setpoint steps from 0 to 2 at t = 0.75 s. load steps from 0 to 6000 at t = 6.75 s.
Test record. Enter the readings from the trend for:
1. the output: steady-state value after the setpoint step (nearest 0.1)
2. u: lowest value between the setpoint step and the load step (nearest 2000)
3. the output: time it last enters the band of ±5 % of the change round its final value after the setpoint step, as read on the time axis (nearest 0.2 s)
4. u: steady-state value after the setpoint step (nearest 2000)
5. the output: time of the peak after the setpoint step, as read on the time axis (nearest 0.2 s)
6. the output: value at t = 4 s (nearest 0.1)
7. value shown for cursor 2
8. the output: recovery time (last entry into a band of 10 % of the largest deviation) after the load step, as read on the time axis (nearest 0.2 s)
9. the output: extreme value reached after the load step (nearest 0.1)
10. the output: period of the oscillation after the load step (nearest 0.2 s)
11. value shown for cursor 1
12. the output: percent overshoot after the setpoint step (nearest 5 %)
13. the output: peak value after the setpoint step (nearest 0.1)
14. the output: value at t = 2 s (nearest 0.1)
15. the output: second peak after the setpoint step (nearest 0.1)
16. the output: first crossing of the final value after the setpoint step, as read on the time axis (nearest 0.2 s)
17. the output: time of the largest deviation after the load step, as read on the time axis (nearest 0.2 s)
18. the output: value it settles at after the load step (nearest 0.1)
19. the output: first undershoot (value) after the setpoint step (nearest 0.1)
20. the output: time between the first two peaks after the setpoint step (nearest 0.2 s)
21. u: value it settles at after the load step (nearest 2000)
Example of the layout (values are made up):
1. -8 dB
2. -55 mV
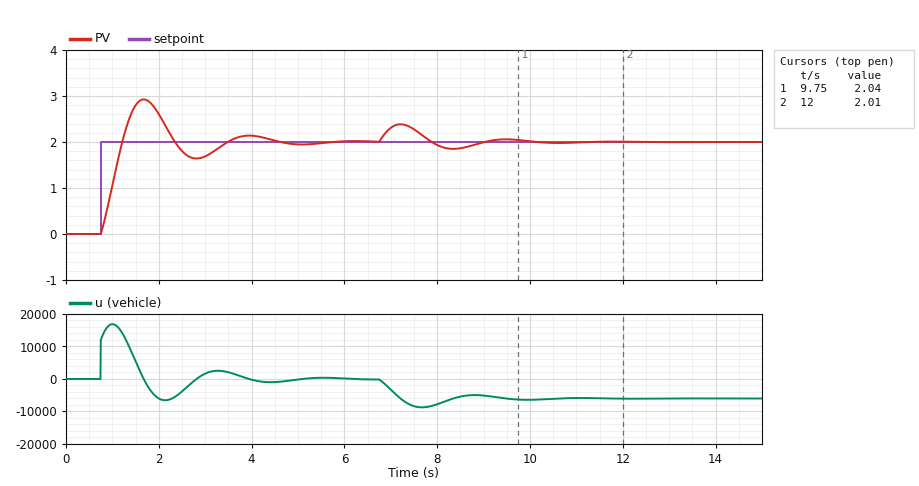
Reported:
1. 2.0
2. -6000
3. 4.2 s
4. 0
5. 1.6 s
6. 2.1
7. 2.01
8. 9.8 s
9. 2.4
10. 2.2 s
11. 2.04
12. 45 %
13. 2.9
14. 2.6
15. 2.1
16. 1.2 s
17. 7.2 s
18. 2.0
19. 1.6
20. 2.2 s
21. -6000
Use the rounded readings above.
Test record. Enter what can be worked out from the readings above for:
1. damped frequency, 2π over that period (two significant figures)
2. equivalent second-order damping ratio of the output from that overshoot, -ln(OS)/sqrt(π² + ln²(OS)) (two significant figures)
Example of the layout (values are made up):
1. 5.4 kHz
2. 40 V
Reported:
1. 2.9 rad/s
2. 0.25
